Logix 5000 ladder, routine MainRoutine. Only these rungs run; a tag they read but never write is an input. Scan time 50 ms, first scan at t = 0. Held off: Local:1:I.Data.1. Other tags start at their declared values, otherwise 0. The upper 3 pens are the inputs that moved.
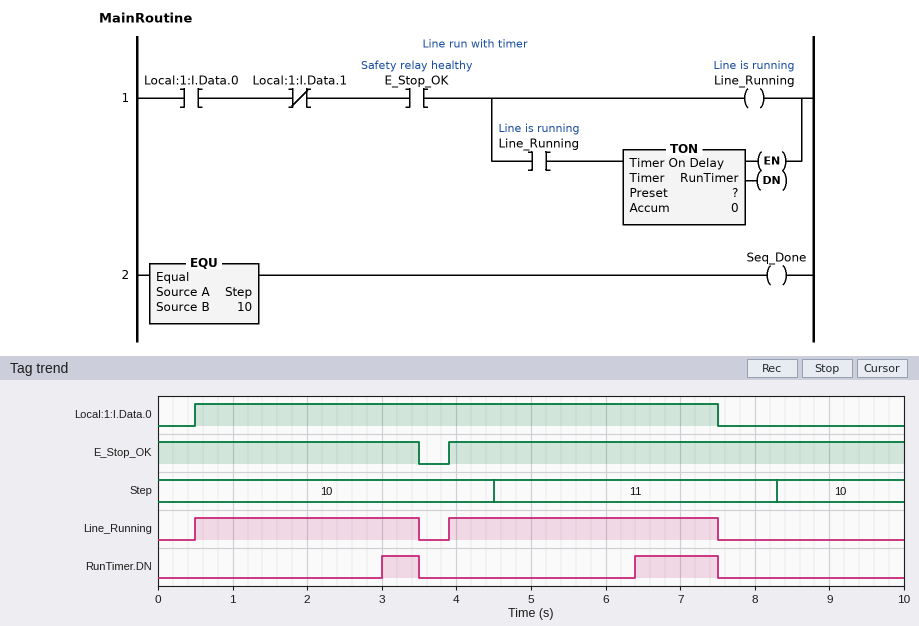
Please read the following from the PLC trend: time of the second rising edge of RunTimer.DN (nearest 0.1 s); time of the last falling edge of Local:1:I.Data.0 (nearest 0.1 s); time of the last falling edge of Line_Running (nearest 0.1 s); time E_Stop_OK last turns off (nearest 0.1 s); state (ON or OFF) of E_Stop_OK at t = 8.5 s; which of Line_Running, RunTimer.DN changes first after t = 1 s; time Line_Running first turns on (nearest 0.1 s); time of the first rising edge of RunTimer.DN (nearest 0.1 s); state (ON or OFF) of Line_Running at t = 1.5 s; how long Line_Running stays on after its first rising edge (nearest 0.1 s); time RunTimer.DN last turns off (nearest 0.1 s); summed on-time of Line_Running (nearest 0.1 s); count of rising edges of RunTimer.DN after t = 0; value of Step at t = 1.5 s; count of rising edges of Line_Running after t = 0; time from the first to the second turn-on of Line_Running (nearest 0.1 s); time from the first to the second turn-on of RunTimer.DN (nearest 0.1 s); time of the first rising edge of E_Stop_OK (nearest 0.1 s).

6.4 s
7.5 s
7.5 s
3.5 s
ON
RunTimer.DN
0.5 s
3.0 s
ON
3.0 s
7.5 s
6.6 s
2
10
2
3.4 s
3.4 s
3.9 s
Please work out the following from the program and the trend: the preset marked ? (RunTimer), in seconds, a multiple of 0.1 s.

2.5 s
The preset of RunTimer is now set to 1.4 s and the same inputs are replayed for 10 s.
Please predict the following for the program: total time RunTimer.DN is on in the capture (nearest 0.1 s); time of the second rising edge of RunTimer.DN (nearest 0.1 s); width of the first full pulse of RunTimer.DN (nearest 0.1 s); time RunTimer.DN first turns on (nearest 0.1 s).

3.8 s
5.3 s
1.6 s
1.9 s
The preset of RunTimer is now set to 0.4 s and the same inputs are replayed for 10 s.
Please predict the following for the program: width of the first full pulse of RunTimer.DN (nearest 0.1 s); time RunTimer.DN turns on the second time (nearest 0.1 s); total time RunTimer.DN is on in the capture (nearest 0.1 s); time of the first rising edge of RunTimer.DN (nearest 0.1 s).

2.6 s
4.3 s
5.8 s
0.9 s
